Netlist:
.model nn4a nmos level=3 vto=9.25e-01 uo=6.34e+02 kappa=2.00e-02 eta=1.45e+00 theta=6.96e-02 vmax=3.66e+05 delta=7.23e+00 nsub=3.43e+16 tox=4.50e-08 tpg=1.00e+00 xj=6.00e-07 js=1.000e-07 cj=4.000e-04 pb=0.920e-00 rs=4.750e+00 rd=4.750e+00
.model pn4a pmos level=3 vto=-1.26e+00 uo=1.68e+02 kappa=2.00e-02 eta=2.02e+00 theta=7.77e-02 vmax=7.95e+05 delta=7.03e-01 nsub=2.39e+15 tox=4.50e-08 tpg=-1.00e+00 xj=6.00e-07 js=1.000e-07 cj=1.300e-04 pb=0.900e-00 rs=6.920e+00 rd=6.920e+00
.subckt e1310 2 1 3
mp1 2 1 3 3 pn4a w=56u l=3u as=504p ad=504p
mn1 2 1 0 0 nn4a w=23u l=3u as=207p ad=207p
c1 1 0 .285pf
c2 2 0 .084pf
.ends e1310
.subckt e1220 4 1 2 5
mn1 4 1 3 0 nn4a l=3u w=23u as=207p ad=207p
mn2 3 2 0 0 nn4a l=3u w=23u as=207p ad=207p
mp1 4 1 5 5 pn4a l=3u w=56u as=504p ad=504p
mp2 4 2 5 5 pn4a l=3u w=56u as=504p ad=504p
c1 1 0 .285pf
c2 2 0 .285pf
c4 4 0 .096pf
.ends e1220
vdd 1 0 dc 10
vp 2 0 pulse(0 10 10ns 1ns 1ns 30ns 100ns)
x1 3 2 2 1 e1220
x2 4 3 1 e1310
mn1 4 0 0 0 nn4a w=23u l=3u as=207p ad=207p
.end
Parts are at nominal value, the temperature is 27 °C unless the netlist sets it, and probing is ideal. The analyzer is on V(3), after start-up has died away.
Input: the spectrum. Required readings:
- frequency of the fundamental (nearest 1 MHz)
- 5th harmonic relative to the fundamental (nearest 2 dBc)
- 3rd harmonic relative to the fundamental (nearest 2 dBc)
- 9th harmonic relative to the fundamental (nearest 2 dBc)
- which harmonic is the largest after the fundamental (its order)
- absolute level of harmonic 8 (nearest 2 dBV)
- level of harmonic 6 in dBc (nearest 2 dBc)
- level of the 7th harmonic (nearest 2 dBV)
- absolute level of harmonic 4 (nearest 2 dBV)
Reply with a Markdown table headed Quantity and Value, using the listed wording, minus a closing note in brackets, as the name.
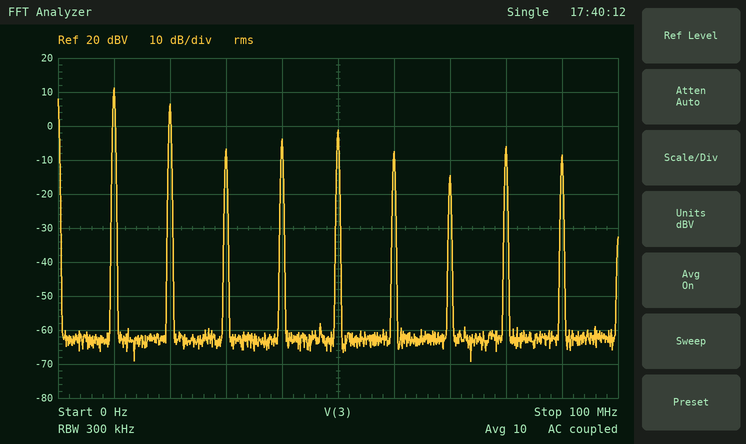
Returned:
| Quantity | Value |
|---|---|
| frequency of the fundamental | 10 MHz |
| 5th harmonic relative to the fundamental | -12 dBc |
| 3rd harmonic relative to the fundamental | -18 dBc |
| 9th harmonic relative to the fundamental | -20 dBc |
| which harmonic is the largest after the fundamental | 2 |
| absolute level of harmonic 8 | -6 dBV |
| level of harmonic 6 in dBc | -18 dBc |
| level of the 7th harmonic | -14 dBV |
| absolute level of harmonic 4 | -4 dBV |
